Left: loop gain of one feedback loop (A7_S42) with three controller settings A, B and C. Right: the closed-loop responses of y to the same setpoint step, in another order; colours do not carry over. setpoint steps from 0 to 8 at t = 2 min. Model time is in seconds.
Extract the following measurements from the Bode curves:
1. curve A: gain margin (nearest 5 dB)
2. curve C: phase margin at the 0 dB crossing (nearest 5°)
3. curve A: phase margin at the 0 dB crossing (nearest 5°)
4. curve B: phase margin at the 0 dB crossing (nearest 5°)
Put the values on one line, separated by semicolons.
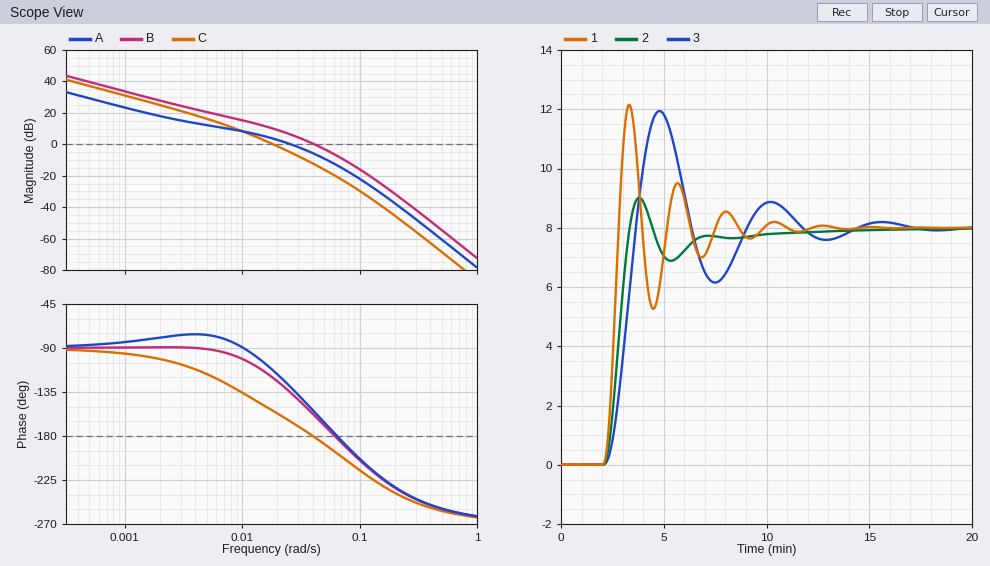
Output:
15 dB; 25°; 50°; 20°
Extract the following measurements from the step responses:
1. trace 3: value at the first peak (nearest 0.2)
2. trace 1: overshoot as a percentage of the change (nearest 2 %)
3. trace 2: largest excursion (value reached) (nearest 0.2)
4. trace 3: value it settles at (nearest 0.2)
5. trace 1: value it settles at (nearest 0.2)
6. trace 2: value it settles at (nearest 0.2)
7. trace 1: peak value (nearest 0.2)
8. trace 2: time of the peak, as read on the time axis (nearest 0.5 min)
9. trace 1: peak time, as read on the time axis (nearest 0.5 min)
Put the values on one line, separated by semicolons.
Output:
12.0; 52 %; 9.0; 8.0; 8.0; 8.0; 12.2; 4.0 min; 3.5 min
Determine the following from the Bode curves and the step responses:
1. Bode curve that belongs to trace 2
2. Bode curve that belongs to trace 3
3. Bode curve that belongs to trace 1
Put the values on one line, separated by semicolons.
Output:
A; C; B
